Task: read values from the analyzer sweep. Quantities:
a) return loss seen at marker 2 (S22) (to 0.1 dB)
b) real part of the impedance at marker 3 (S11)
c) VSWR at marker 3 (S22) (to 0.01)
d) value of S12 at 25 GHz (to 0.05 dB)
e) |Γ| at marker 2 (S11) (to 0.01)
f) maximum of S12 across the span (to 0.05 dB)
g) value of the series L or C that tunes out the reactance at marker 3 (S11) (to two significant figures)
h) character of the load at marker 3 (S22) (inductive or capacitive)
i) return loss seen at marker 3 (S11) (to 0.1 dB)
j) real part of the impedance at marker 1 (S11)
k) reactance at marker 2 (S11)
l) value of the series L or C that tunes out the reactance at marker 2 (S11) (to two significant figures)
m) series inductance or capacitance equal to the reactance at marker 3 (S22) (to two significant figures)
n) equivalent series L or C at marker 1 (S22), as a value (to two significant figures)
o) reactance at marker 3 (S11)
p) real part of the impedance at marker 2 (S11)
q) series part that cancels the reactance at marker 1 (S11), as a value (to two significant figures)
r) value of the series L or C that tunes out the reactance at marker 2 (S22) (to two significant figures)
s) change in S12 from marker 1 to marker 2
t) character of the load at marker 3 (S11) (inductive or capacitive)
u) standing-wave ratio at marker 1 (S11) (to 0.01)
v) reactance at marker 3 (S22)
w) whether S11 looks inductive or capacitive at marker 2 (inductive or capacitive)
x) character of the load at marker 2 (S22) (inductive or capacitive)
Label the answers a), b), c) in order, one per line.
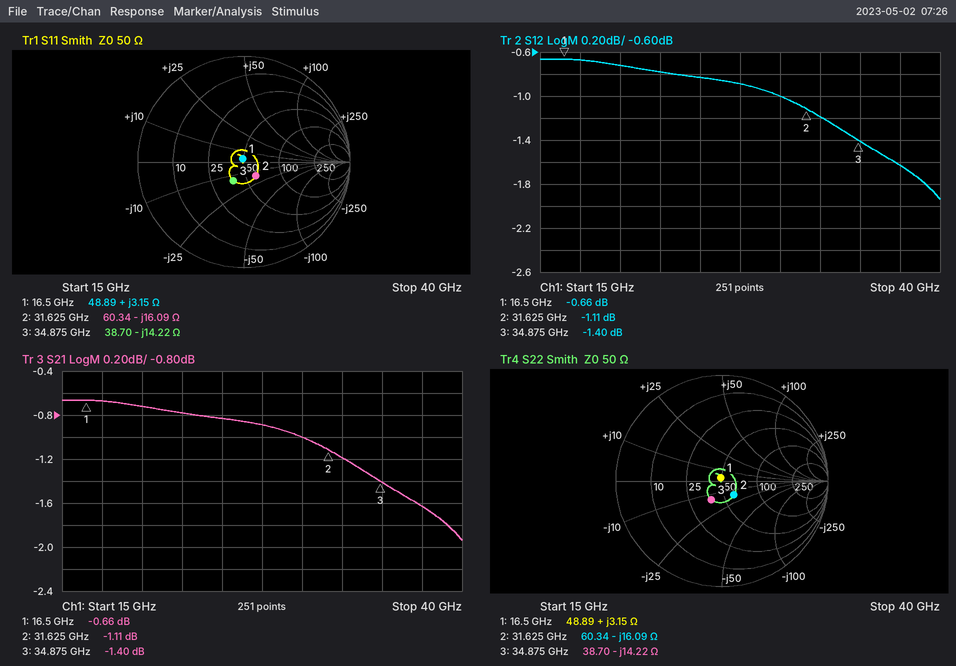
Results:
a) 15.3 dB
b) 38.70 Ω
c) 1.51
d) -0.85 dB
e) 0.17
f) -0.65 dB
g) 65 pH
h) capacitive
i) 13.9 dB
j) 48.89 Ω
k) -16.09 Ω
l) 81 pH
m) 320 fF
n) 30 pH
o) -14.22 Ω
p) 60.34 Ω
q) 3.1 pF
r) 81 pH
s) -0.45 dB
t) capacitive
u) 1.07
v) -14.22 Ω
w) capacitive
x) capacitive
